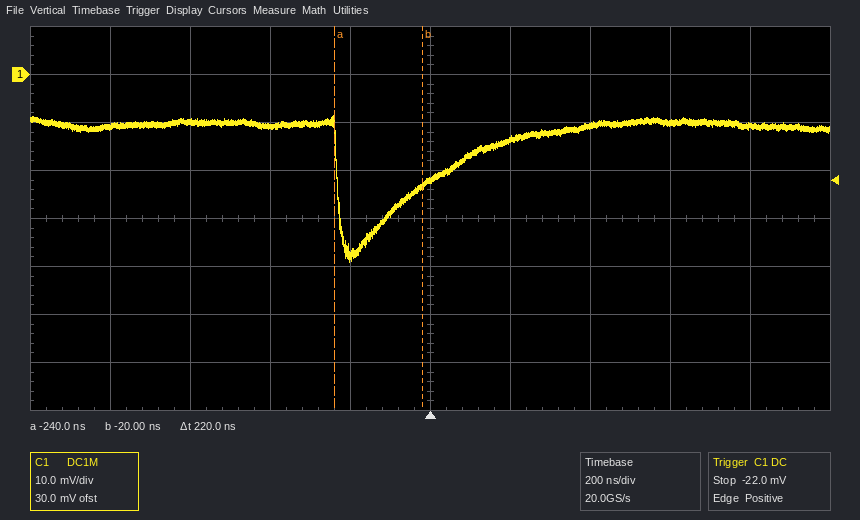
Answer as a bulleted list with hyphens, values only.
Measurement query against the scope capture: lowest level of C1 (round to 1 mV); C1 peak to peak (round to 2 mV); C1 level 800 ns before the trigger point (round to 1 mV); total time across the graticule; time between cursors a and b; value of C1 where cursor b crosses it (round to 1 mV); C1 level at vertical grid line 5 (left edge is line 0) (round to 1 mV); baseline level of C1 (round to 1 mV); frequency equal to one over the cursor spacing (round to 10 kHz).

- -39 mV
- 30 mV
- -11 mV
- 2 µs
- 220 ns
- -23 mV
- -22 mV
- -10 mV
- 4.55 MHz
